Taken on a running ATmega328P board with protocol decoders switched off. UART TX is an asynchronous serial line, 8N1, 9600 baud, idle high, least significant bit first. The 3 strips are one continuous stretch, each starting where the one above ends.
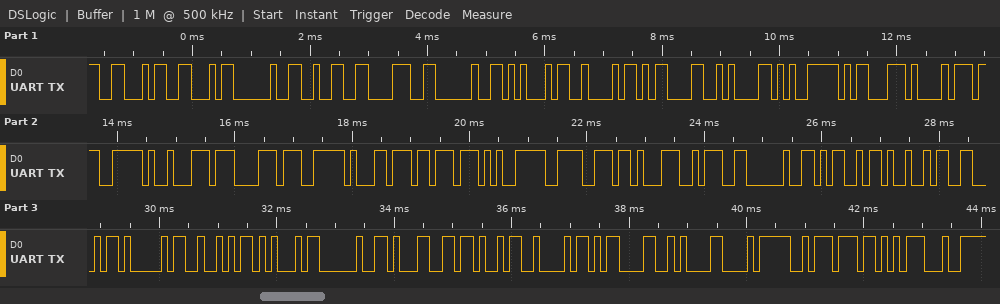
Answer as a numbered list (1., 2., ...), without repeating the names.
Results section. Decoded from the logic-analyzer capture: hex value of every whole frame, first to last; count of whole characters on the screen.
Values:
1. 0x46 0x46 0x20 0x32 0x38 0x20 0x45 0x42 0x0D 0x0A 0xE5 0x8D 0xA1 0xE7 0x89 0x87 0xE7 0xB1 0xBB 0xE5 0x9E 0x8B 0x3A 0x20 0x4D 0x49 0x46 0x41 0x52 0x45 0x20 0x31 0x4B 0x42 0x0D 0x0A 0xE8 0xBA 0xAB 0xE4
2. 40
